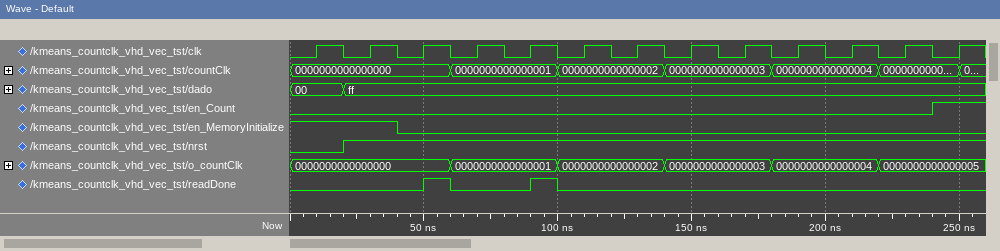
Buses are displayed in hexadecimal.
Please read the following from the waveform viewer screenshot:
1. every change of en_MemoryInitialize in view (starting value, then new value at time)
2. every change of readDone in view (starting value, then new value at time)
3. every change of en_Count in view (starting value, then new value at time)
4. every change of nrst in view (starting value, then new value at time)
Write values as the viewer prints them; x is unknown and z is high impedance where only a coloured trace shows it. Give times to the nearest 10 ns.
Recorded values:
1, 0 at 40 ns
0, 1 at 50 ns, 0 at 60 ns, 1 at 90 ns, 0 at 100 ns
0, 1 at 240 ns
0, 1 at 20 ns
